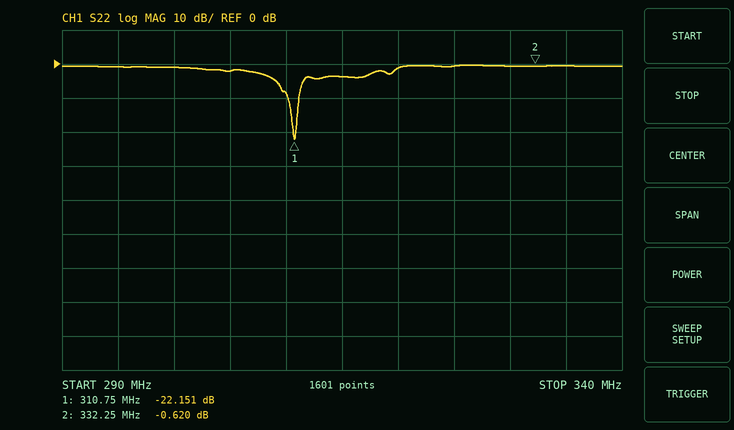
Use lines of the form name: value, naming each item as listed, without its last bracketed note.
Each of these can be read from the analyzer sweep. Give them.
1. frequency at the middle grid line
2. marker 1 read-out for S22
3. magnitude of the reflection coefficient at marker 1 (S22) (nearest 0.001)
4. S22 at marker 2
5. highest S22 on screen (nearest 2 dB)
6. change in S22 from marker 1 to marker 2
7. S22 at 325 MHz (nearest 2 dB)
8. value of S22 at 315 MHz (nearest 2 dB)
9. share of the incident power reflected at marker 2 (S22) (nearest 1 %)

frequency at the middle grid line: 315 MHz
marker 1 read-out for S22: -22.151 dB
magnitude of the reflection coefficient at marker 1 (S22): 0.078
S22 at marker 2: -0.620 dB
highest S22 on screen: 0 dB
change in S22 from marker 1 to marker 2: 21.531 dB
S22 at 325 MHz: 0 dB
value of S22 at 315 MHz: -4 dB
share of the incident power reflected at marker 2 (S22): 87 %
